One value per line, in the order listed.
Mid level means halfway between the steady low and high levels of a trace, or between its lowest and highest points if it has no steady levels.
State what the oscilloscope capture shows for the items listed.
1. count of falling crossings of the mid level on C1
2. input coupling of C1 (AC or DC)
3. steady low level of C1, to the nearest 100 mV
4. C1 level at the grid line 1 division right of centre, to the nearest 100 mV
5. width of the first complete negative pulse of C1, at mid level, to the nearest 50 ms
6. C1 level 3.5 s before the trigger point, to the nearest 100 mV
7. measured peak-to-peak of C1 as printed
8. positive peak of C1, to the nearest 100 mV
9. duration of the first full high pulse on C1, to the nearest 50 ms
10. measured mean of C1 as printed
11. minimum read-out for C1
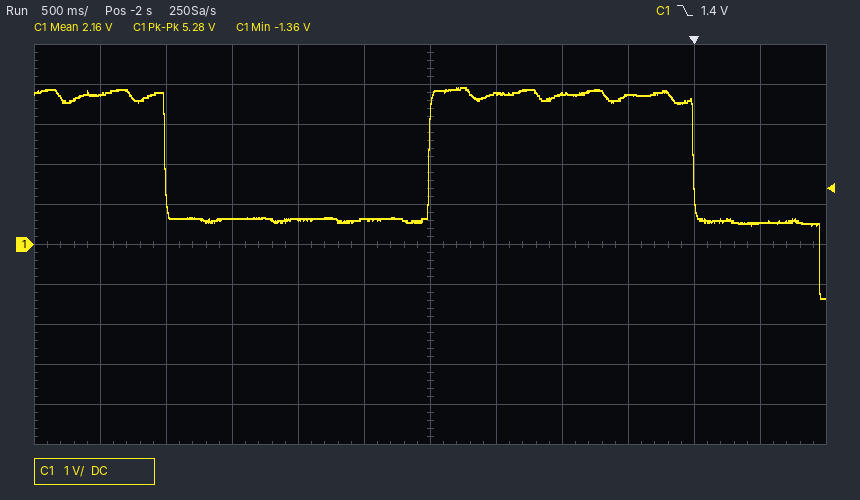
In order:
2
DC
600 mV
3.8 V
2.00 s
600 mV
5.28 V
3.9 V
2.00 s
2.16 V
-1.36 V
